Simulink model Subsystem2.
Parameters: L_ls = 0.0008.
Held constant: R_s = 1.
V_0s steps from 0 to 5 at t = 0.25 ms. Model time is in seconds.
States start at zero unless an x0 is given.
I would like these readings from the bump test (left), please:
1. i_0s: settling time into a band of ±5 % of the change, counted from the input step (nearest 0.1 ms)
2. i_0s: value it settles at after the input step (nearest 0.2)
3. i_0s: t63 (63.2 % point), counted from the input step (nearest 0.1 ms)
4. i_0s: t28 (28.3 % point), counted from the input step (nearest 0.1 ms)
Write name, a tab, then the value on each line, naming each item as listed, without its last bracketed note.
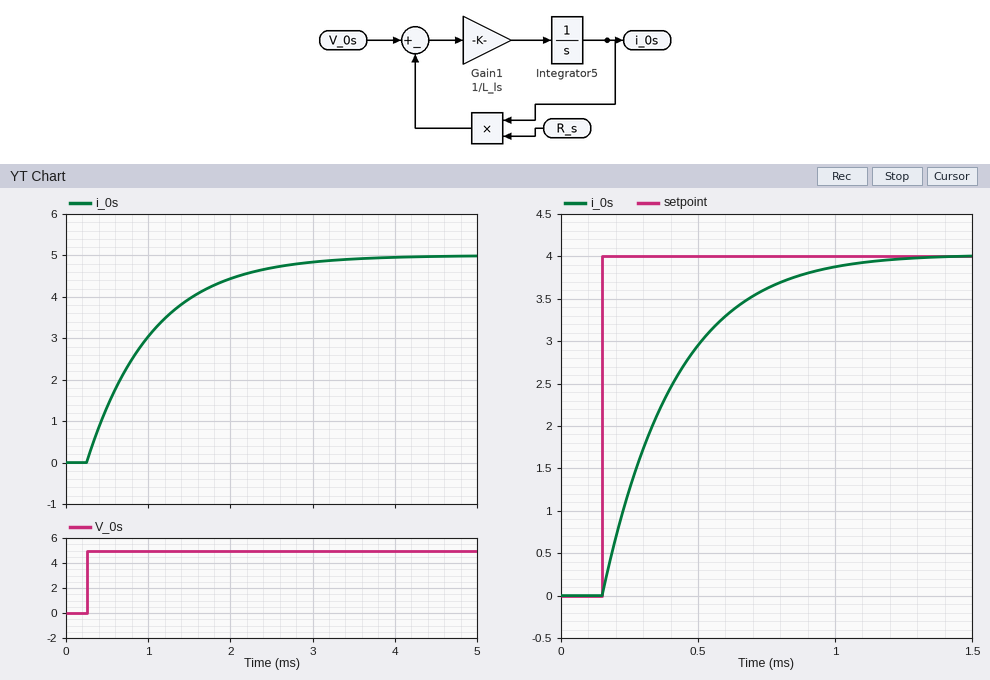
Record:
i_0s: settling time into a band of ±5 % of the change, counted from the input step	2.4 ms
i_0s: value it settles at after the input step	5.0
i_0s: t63 (63.2 % point), counted from the input step	0.8 ms
i_0s: t28 (28.3 % point), counted from the input step	0.3 ms
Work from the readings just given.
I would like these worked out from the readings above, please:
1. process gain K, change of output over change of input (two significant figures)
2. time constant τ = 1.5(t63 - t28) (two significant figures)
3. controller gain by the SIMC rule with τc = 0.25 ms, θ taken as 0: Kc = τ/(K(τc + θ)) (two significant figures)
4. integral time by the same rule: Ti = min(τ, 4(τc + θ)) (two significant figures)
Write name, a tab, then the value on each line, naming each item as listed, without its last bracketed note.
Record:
process gain K, change of output over change of input	1.0
time constant τ = 1.5(t63 - t28)	0.75 ms
controller gain by the SIMC rule with τc = 0.25 ms, θ taken as 0: Kc = τ/(K(τc + θ))	3.0
integral time by the same rule: Ti = min(τ, 4(τc + θ))	0.75 ms
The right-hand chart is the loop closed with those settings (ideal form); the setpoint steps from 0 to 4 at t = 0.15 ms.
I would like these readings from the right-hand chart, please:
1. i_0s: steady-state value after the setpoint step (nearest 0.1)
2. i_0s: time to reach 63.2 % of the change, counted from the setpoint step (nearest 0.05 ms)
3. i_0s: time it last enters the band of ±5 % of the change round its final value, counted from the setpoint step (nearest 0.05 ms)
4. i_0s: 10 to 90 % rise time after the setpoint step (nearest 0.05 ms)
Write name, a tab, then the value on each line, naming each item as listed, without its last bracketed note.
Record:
i_0s: steady-state value after the setpoint step	4.0
i_0s: time to reach 63.2 % of the change, counted from the setpoint step	0.25 ms
i_0s: time it last enters the band of ±5 % of the change round its final value, counted from the setpoint step	0.75 ms
i_0s: 10 to 90 % rise time after the setpoint step	0.55 ms
